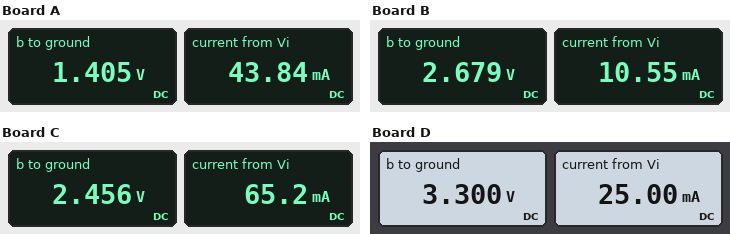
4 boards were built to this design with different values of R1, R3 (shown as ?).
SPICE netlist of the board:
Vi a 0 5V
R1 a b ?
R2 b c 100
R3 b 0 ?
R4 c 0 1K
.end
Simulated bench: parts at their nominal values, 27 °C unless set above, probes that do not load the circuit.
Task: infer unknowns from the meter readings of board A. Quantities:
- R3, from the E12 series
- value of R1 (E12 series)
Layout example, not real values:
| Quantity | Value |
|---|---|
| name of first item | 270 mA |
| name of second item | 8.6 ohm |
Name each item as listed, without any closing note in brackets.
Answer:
| Quantity | Value |
|---|---|
| R3, from the E12 series | 33 Ω |
| value of R1 | 82 Ω |
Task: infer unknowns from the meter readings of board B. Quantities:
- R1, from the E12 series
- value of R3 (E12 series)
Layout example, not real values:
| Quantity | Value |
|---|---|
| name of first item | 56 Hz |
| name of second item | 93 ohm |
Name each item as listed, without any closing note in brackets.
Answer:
| Quantity | Value |
|---|---|
| R1, from the E12 series | 220 Ω |
| value of R3 | 330 Ω |
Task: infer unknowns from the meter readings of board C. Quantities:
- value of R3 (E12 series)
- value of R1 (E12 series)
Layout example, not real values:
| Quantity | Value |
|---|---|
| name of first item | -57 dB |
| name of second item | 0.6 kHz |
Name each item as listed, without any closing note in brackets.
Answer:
| Quantity | Value |
|---|---|
| value of R3 | 39 Ω |
| value of R1 | 39 Ω |
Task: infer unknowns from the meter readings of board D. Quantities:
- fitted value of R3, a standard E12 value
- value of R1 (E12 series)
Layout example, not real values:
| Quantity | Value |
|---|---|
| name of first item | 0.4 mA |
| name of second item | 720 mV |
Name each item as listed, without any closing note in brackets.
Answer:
| Quantity | Value |
|---|---|
| fitted value of R3, a standard E12 value | 150 Ω |
| value of R1 | 68 Ω |
